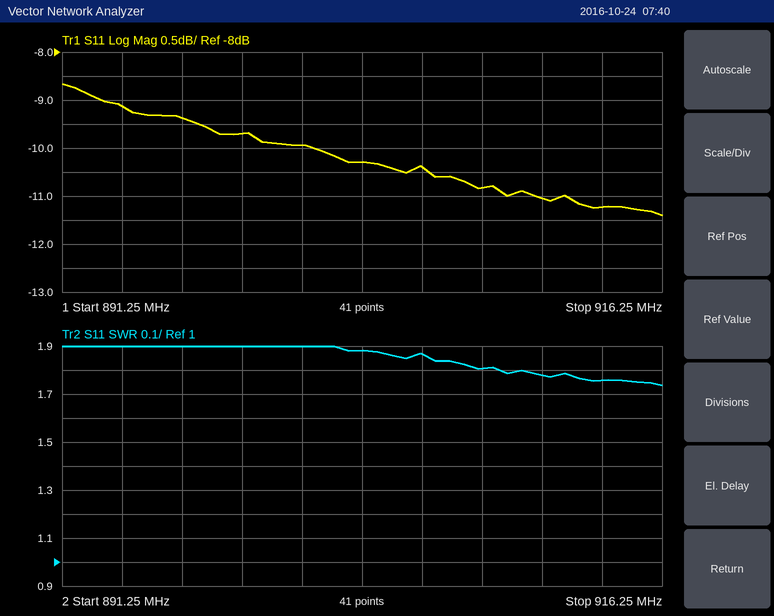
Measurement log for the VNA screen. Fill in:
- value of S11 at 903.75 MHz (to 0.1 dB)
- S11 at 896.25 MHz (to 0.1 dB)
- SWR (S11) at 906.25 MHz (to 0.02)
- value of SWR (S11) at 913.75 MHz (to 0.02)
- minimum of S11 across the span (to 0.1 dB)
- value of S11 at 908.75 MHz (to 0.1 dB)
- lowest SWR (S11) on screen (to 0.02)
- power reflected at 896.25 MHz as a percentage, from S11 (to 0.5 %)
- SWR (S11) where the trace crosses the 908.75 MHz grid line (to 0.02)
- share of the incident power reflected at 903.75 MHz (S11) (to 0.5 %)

-10.3 dB
-9.4 dB
1.86
1.76
-11.4 dB
-10.8 dB
1.74
11.5 %
1.80
9.5 %
